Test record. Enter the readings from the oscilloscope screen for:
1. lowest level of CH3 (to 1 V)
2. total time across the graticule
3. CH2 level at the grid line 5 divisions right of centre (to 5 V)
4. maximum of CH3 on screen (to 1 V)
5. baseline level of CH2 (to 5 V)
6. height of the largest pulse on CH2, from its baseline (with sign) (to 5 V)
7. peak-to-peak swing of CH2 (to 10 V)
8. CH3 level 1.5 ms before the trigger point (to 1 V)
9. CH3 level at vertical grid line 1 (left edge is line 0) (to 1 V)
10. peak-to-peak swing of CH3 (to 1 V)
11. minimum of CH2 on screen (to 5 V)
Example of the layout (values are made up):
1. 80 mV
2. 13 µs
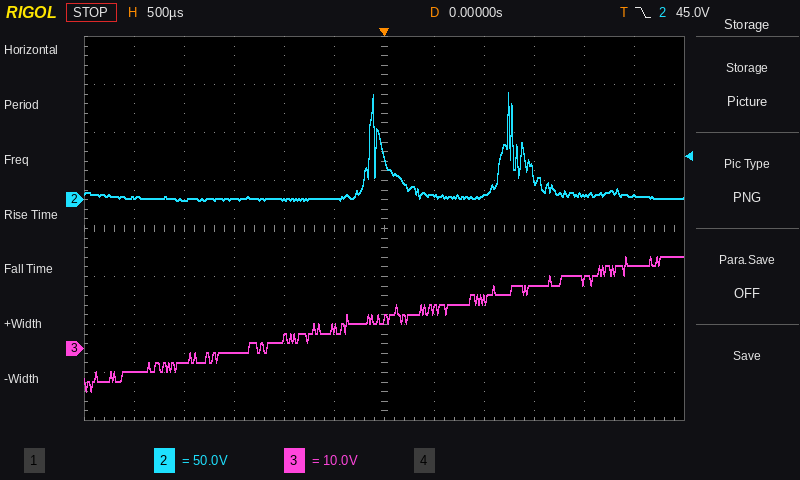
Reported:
1. -9 V
2. 6 ms
3. 5 V
4. 19 V
5. 0 V
6. +110 V
7. 110 V
8. -1 V
9. -5 V
10. 28 V
11. 0 V
